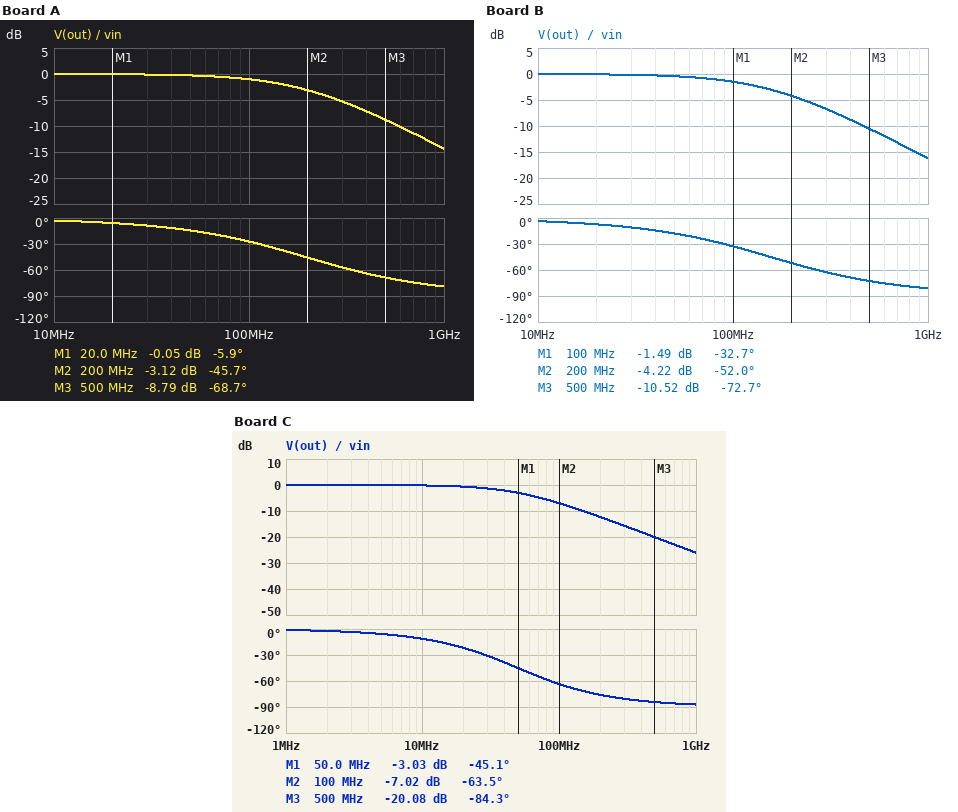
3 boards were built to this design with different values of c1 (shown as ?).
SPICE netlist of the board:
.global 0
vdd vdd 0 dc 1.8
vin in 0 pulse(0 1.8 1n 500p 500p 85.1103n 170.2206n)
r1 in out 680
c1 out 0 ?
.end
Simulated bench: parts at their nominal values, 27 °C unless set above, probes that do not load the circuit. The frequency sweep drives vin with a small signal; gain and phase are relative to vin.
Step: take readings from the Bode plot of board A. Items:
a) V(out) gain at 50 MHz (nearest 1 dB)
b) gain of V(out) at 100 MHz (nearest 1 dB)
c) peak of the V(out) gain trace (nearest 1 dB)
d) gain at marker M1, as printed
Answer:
0 dB
-1 dB
0 dB
-0.05 dB
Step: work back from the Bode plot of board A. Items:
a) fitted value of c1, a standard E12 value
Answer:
1.2 pF
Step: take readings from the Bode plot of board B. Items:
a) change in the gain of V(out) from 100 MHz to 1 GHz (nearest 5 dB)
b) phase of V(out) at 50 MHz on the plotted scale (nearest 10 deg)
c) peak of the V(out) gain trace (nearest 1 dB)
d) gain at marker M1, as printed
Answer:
-15 dB
-20 deg
0 dB
-1.49 dB
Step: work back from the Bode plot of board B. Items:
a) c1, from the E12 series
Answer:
1.5 pF
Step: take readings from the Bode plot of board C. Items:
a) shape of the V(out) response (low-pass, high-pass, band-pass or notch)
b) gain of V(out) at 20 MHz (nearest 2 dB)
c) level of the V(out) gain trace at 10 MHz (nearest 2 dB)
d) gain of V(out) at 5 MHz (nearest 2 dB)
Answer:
low-pass
0 dB
0 dB
0 dB
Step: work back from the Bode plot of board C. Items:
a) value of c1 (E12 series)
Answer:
4.7 pF
